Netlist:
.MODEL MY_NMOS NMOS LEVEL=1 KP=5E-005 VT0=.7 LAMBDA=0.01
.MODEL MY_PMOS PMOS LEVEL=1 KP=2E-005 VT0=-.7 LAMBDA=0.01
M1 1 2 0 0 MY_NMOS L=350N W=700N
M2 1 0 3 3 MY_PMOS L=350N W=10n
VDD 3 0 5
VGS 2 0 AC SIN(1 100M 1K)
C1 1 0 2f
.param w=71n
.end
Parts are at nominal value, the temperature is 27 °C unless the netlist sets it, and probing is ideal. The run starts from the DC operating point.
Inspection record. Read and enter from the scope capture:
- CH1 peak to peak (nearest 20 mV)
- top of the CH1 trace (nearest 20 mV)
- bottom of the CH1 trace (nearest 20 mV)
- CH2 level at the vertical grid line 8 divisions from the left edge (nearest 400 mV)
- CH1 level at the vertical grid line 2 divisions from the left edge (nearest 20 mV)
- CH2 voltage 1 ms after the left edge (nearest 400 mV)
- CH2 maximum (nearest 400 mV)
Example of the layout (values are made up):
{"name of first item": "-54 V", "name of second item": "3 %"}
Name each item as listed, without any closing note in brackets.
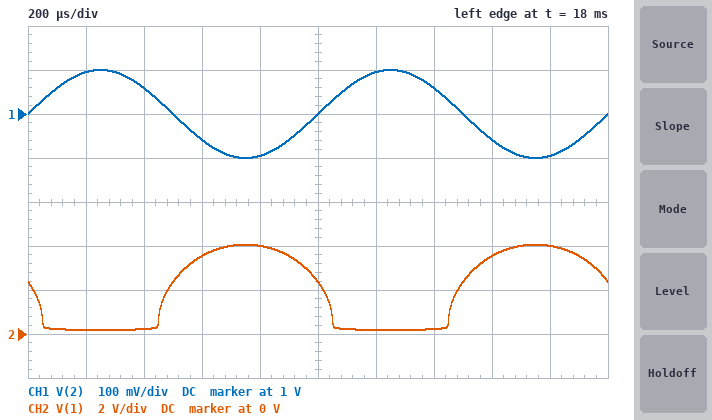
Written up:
{"CH1 peak to peak": "200 mV", "top of the CH1 trace": "1.10 V", "bottom of the CH1 trace": "900 mV", "CH2 level at the vertical grid line 8 divisions from the left edge": "3.6 V", "CH1 level at the vertical grid line 2 divisions from the left edge": "1.06 V", "CH2 voltage 1 ms after the left edge": "2.4 V", "CH2 maximum": "4.0 V"}
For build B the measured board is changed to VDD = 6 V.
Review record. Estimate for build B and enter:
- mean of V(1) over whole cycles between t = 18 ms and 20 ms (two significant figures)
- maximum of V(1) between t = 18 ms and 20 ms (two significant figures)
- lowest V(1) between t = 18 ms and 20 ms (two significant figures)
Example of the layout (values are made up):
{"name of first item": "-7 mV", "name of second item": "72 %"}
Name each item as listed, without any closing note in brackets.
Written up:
{"mean of V(1) over whole cycles between t = 18 ms and 20 ms": "3.8 V", "maximum of V(1) between t = 18 ms and 20 ms": "5.3 V", "lowest V(1) between t = 18 ms and 20 ms": "1.6 V"}
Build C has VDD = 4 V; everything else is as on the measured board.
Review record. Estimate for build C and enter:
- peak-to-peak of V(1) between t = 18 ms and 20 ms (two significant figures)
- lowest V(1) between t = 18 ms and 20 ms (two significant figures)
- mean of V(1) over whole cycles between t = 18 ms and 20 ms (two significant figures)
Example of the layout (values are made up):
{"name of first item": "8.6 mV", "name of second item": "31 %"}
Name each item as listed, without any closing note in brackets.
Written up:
{"peak-to-peak of V(1) between t = 18 ms and 20 ms": "2.6 V", "lowest V(1) between t = 18 ms and 20 ms": "91 mV", "mean of V(1) over whole cycles between t = 18 ms and 20 ms": "840 mV"}
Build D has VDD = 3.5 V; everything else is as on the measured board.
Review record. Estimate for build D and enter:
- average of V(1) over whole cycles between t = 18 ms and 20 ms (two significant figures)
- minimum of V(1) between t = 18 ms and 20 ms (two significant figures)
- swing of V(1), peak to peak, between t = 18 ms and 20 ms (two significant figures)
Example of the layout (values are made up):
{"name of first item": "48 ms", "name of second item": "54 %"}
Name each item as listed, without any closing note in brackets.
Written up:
{"average of V(1) over whole cycles between t = 18 ms and 20 ms": "320 mV", "minimum of V(1) between t = 18 ms and 20 ms": "63 mV", "swing of V(1), peak to peak, between t = 18 ms and 20 ms": "1.6 V"}
